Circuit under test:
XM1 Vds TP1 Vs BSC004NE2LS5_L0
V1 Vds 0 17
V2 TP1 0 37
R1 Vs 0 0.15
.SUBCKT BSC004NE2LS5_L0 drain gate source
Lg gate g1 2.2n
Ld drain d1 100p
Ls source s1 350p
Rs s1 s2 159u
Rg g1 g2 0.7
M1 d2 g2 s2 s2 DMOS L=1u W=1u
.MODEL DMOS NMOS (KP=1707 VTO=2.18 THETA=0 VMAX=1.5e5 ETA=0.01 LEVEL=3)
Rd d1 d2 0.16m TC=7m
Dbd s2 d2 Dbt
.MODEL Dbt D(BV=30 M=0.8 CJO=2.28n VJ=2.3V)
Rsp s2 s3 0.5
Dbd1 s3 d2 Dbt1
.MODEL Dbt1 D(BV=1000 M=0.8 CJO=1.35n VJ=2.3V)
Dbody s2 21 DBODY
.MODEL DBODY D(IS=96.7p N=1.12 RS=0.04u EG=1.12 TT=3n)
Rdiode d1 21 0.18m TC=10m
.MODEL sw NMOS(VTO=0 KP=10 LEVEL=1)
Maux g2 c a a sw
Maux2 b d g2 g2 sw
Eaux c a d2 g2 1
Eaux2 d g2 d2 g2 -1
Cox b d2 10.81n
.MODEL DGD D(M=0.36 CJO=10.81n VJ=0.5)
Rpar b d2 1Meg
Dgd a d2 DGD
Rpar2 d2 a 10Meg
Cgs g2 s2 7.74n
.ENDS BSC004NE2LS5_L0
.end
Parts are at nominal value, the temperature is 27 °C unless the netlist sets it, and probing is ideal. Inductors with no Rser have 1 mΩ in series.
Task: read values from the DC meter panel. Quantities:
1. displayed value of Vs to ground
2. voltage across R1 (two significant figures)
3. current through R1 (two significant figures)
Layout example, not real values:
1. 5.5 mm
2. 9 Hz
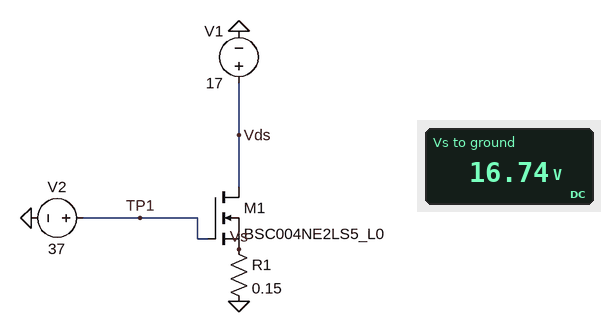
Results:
1. 16.74 V
2. 17 V
3. 110 A
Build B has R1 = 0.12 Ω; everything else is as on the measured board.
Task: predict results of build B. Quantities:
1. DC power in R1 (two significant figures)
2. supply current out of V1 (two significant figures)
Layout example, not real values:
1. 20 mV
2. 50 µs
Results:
1. 2.3 kW
2. 140 A
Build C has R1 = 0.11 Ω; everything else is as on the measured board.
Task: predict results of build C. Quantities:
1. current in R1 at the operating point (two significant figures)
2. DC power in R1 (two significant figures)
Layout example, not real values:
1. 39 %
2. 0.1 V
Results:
1. 150 A
2. 2.5 kW
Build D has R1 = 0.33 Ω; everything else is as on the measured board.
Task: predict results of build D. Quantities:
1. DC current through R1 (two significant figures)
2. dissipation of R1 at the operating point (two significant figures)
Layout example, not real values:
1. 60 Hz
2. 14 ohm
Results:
1. 51 A
2. 860 W
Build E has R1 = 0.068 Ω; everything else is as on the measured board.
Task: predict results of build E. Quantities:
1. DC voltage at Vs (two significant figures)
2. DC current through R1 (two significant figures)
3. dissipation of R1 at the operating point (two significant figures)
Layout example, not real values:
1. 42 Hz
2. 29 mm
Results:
1. 16 V
2. 240 A
3. 4.0 kW
